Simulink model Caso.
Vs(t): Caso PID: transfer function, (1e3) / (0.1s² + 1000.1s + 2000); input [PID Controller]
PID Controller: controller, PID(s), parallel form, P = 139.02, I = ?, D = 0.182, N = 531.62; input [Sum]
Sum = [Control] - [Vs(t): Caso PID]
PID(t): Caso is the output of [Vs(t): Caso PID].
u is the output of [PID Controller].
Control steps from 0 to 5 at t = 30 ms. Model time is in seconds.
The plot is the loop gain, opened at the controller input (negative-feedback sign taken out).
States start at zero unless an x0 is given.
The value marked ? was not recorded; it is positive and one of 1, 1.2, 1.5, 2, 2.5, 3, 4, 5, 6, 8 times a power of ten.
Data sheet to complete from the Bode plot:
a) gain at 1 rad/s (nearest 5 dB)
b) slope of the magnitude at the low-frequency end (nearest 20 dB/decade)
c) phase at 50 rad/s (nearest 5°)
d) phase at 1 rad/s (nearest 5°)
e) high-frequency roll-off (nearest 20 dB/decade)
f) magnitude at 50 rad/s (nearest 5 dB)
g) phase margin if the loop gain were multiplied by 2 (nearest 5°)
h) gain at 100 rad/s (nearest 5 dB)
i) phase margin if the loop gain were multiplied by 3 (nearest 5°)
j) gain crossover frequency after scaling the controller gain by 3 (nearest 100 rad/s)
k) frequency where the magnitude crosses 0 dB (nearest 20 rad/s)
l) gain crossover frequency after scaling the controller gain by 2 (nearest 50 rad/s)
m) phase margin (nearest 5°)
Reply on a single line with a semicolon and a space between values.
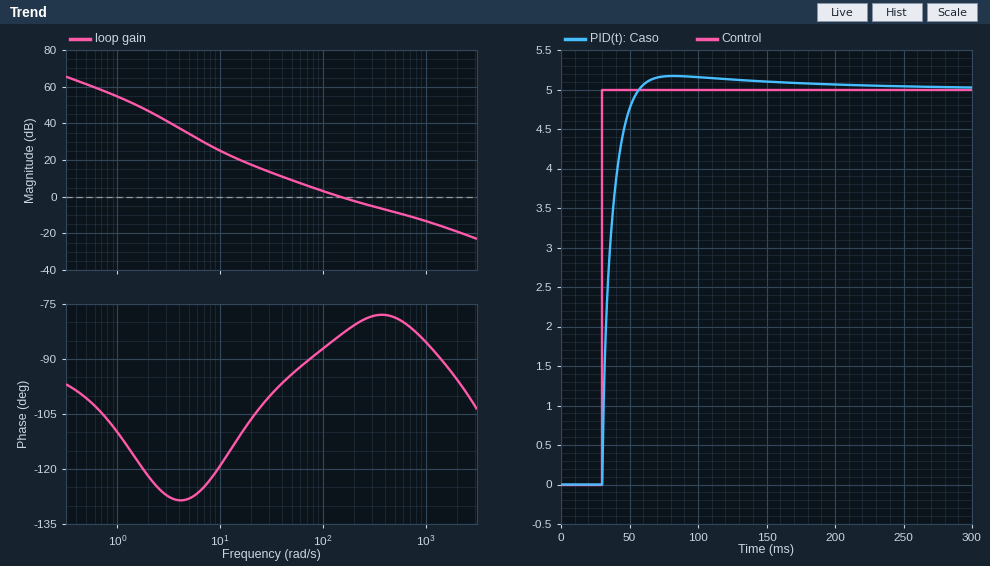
55 dB; -20 dB/decade; -95°; -110°; -20 dB/decade; 10 dB; 100°; 5 dB; 100°; 600 rad/s; 140 rad/s; 350 rad/s; 95°
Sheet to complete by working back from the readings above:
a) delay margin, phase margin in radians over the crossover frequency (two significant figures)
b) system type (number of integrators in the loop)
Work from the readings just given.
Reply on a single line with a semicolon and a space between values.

0.012 s; 1
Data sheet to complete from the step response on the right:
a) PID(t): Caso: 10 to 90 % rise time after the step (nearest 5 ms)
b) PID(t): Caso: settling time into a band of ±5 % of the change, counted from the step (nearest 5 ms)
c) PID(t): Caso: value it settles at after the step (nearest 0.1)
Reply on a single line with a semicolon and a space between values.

15 ms; 20 ms; 5.0
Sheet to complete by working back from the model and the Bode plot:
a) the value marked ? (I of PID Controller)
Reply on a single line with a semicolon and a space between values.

1200
